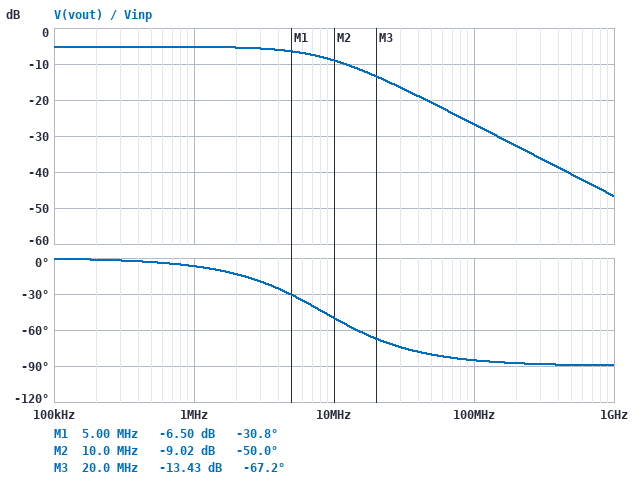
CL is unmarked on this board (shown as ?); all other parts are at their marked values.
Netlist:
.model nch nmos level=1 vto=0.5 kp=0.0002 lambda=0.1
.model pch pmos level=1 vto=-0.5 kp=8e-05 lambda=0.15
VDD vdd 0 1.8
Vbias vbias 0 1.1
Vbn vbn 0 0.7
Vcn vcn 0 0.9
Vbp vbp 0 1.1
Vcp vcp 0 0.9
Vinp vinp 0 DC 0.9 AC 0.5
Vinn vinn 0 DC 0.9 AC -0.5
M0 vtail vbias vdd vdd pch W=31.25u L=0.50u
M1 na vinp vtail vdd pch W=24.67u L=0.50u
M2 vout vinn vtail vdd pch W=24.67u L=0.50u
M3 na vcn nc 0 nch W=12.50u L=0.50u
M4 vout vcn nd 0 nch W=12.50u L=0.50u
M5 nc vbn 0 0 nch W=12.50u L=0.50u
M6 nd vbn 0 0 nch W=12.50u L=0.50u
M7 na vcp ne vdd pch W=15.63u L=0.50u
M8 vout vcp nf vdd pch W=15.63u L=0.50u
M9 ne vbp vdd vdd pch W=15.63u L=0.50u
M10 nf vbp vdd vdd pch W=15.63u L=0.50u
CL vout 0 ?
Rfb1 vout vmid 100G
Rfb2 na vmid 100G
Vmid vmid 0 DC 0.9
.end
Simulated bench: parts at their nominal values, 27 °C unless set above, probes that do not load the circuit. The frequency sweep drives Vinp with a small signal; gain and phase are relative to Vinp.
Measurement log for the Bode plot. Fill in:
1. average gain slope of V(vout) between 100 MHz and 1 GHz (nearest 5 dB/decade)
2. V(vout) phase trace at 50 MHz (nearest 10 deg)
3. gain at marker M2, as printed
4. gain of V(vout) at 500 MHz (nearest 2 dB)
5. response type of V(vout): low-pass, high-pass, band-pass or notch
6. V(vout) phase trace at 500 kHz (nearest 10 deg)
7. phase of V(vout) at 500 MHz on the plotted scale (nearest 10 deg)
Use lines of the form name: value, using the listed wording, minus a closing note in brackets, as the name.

average gain slope of V(vout) between 100 MHz and 1 GHz: -20 dB/decade
V(vout) phase trace at 50 MHz: -80 deg
gain at marker M2, as printed: -9.02 dB
gain of V(vout) at 500 MHz: -40 dB
response type of V(vout): low-pass, high-pass, band-pass or notch: low-pass
V(vout) phase trace at 500 kHz: 0 deg
phase of V(vout) at 500 MHz on the plotted scale: -90 deg
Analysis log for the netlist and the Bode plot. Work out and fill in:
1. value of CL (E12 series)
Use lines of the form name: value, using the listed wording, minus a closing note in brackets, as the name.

value of CL: 1.2 pF
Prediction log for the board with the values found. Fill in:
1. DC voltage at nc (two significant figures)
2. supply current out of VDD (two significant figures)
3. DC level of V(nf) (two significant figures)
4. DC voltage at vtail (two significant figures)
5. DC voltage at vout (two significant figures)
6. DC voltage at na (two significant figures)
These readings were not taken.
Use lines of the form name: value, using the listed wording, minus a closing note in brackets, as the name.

DC voltage at nc: 210 mV
supply current out of VDD: 200 µA
DC level of V(nf): 1.6 V
DC voltage at vtail: 1.6 V
DC voltage at vout: 1.5 V
DC voltage at na: 1.5 V
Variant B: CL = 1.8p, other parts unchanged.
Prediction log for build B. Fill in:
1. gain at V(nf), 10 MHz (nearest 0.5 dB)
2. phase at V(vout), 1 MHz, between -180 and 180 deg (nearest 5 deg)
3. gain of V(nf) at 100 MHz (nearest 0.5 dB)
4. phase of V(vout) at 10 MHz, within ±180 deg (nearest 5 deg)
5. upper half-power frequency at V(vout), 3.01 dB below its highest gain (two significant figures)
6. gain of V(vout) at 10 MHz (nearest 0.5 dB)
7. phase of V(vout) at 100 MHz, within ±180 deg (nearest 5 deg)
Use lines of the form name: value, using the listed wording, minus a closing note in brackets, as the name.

gain at V(nf), 10 MHz: -19.0 dB
phase at V(vout), 1 MHz, between -180 and 180 deg: -10 deg
gain of V(nf) at 100 MHz: -38.0 dB
phase of V(vout) at 10 MHz, within ±180 deg: -60 deg
upper half-power frequency at V(vout), 3.01 dB below its highest gain: 5.6 MHz
gain of V(vout) at 10 MHz: -11.5 dB
phase of V(vout) at 100 MHz, within ±180 deg: -85 deg
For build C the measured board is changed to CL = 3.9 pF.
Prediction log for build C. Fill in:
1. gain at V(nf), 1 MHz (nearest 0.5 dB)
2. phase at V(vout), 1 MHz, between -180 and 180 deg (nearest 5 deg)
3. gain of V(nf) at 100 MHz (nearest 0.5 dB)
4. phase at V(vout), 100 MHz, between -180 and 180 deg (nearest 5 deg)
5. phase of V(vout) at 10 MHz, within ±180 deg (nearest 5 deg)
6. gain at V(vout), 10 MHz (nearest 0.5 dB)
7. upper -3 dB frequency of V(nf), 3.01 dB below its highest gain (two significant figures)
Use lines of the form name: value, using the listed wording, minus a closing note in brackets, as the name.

gain at V(nf), 1 MHz: -13.5 dB
phase at V(vout), 1 MHz, between -180 and 180 deg: -20 deg
gain of V(nf) at 100 MHz: -44.5 dB
phase at V(vout), 100 MHz, between -180 and 180 deg: -90 deg
phase of V(vout) at 10 MHz, within ±180 deg: -75 deg
gain at V(vout), 10 MHz: -17.0 dB
upper -3 dB frequency of V(nf), 3.01 dB below its highest gain: 2.6 MHz
